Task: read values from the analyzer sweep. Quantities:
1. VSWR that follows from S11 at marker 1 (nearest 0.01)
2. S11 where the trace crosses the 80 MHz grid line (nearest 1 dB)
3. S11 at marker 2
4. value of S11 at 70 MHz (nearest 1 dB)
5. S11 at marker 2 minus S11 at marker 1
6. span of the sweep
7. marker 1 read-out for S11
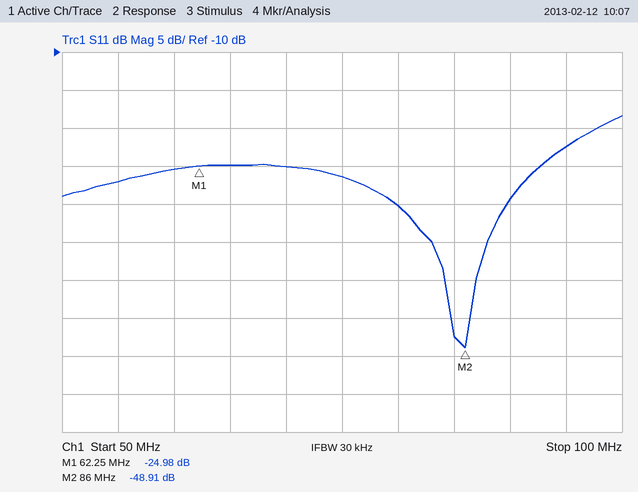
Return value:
1.12
-30 dB
-48.91 dB
-25 dB
-23.93 dB
50 MHz
-24.98 dB
